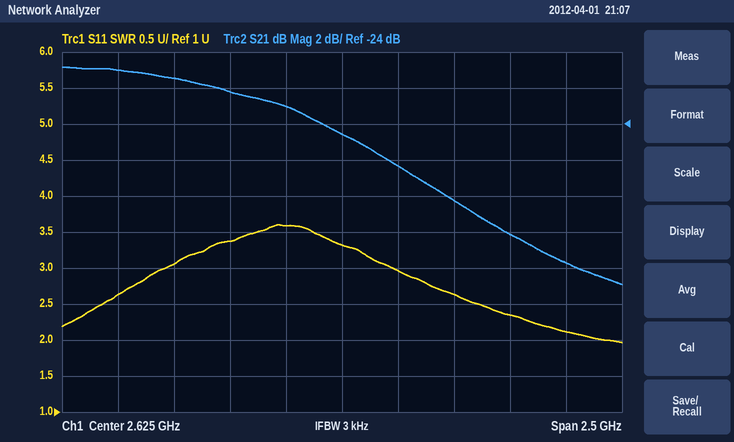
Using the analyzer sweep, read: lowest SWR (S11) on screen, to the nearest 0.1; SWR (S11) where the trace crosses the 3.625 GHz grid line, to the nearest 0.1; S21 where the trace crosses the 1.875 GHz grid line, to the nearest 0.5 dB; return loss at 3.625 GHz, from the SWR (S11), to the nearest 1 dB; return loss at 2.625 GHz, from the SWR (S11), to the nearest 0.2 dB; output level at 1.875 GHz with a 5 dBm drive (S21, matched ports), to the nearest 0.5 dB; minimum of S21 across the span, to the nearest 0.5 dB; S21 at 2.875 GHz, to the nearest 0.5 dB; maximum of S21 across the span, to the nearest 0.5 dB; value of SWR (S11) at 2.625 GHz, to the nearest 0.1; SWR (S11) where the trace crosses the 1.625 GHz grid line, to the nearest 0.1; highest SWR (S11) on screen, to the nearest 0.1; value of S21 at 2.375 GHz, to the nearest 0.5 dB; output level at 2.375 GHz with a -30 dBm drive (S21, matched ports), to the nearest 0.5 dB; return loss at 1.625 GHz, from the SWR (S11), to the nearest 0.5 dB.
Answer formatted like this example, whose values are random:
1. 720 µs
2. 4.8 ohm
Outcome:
1. 2.0
2. 2.1
3. -21.5 dB
4. 9 dB
5. 5.4 dB
6. -16.5 dBm
7. -33.0 dB
8. -26.5 dB
9. -21.0 dB
10. 3.3
11. 2.6
12. 3.6
13. -23.0 dB
14. -53.0 dBm
15. 7.0 dB
